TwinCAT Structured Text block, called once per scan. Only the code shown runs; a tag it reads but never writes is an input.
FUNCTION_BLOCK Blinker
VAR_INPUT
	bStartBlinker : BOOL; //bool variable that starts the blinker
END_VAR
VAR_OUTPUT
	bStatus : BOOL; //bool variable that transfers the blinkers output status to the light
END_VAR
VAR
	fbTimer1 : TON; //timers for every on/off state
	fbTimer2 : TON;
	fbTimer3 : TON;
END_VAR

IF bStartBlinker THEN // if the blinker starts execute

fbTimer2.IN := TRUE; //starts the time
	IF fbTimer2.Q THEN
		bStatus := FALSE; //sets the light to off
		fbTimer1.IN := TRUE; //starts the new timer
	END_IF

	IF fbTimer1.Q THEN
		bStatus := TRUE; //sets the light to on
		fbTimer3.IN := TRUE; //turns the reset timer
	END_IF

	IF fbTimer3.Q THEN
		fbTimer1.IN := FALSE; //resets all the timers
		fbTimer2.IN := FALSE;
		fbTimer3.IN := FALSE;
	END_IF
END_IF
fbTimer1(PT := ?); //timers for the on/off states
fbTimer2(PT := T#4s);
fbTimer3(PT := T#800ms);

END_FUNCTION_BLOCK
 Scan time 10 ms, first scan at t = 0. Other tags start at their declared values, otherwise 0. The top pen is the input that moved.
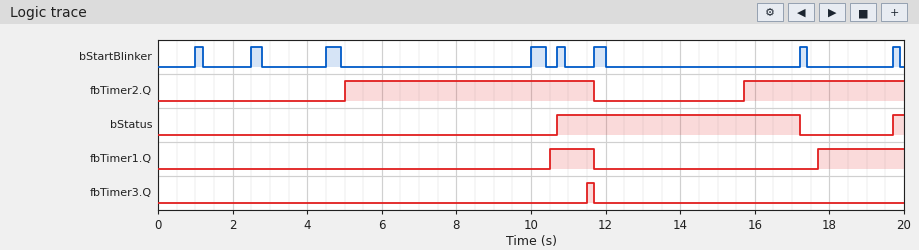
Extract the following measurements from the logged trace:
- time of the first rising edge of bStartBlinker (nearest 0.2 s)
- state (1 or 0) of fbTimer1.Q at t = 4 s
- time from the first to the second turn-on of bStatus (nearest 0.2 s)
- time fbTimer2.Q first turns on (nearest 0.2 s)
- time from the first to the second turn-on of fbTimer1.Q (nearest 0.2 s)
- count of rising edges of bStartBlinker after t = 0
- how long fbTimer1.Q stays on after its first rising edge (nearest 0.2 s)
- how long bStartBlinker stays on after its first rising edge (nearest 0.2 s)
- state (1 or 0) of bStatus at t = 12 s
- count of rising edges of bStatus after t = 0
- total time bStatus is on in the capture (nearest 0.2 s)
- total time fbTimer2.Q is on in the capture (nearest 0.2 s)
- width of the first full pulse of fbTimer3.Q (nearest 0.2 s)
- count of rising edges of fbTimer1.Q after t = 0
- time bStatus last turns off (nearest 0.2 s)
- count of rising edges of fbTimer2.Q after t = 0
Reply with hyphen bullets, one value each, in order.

- 1.0 s
- 0
- 9.0 s
- 5.0 s
- 7.2 s
- 8
- 1.2 s
- 0.2 s
- 1
- 2
- 6.8 s
- 11.0 s
- 0.2 s
- 2
- 17.2 s
- 2
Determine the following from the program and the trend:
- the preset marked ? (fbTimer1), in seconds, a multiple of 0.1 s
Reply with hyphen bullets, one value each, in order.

- 0.5 s
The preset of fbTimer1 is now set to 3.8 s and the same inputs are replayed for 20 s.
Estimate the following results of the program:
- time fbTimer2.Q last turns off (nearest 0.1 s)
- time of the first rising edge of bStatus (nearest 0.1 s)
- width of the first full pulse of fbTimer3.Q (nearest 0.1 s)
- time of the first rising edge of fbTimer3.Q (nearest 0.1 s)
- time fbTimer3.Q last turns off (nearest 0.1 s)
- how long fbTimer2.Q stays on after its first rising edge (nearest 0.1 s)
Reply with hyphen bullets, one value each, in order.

- 19.7 s
- 17.2 s
- 1.7 s
- 18.0 s
- 19.7 s
- 14.7 s
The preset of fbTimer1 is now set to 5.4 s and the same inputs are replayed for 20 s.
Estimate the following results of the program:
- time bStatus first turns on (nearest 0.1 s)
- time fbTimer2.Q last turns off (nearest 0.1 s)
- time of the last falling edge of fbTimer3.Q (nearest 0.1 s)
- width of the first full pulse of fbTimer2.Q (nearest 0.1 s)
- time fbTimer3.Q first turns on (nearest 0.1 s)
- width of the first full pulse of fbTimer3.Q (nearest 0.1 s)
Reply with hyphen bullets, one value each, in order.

- 17.2 s
- 19.7 s
- 19.7 s
- 14.7 s
- 18.0 s
- 1.7 s
